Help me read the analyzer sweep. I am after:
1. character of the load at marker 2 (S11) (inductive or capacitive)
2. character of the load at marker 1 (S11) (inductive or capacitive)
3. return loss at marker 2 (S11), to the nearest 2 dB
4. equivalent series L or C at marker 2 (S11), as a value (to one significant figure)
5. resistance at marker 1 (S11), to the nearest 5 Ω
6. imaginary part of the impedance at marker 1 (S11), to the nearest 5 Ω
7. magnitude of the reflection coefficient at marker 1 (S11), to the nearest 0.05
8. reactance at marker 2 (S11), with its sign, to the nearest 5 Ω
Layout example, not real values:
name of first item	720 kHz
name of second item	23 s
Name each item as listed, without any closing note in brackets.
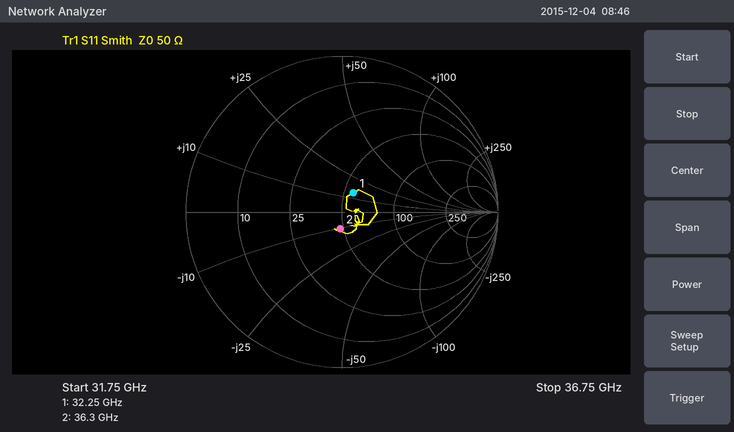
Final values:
character of the load at marker 2 (S11)	capacitive
character of the load at marker 1 (S11)	inductive
return loss at marker 2 (S11), to the nearest 2 dB	20 dB
equivalent series L or C at marker 2 (S11), as a value	400 fF
resistance at marker 1 (S11), to the nearest 5 Ω	55 Ω
imaginary part of the impedance at marker 1 (S11), to the nearest 5 Ω	+15 Ω
magnitude of the reflection coefficient at marker 1 (S11), to the nearest 0.05	0.15
reactance at marker 2 (S11), with its sign, to the nearest 5 Ω	-10 Ω
